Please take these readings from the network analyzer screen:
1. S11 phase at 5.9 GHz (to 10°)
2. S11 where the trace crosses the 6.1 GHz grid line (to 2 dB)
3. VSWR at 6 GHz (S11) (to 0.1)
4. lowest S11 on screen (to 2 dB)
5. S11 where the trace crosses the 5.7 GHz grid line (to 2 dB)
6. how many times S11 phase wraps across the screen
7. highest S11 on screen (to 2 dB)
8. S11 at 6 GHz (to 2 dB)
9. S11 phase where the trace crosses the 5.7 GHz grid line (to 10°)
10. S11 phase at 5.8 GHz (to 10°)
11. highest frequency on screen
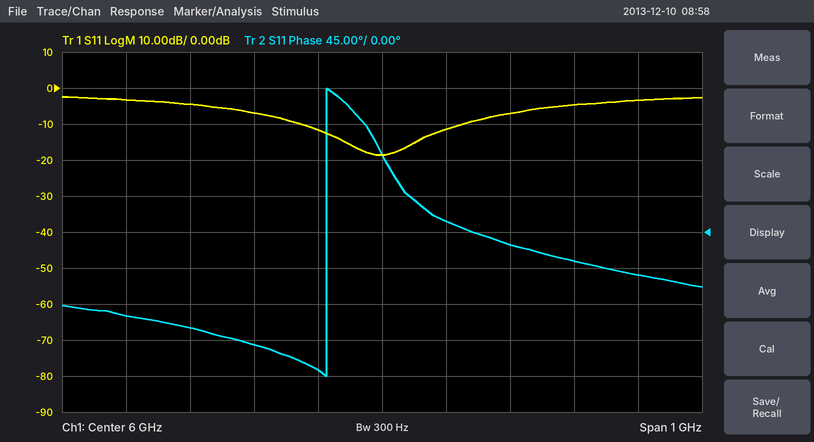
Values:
-170°
-12 dB
1.3
-18 dB
-4 dB
1
-2 dB
-18 dB
-120°
-140°
6.5 GHz
